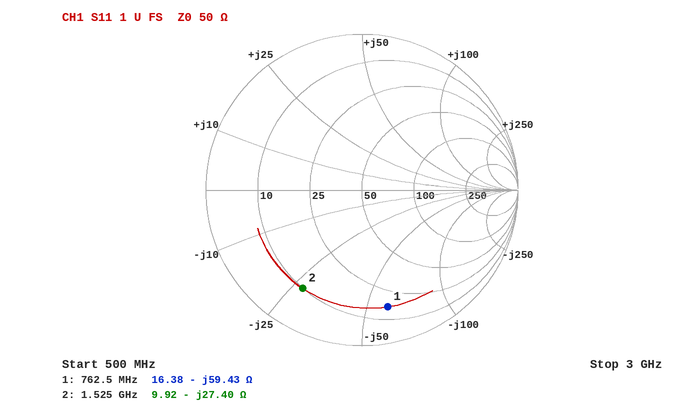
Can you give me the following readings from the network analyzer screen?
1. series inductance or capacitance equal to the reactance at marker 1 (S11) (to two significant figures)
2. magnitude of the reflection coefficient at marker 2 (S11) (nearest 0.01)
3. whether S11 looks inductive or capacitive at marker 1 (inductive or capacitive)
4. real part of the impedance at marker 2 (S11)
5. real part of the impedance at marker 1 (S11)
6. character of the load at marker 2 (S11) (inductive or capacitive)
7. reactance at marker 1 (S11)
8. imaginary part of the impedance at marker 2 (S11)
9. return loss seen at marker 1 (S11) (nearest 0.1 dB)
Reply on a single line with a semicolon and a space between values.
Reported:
3.5 pF; 0.74; capacitive; 9.92 Ω; 16.38 Ω; capacitive; -59.43 Ω; -27.40 Ω; 2.3 dB
